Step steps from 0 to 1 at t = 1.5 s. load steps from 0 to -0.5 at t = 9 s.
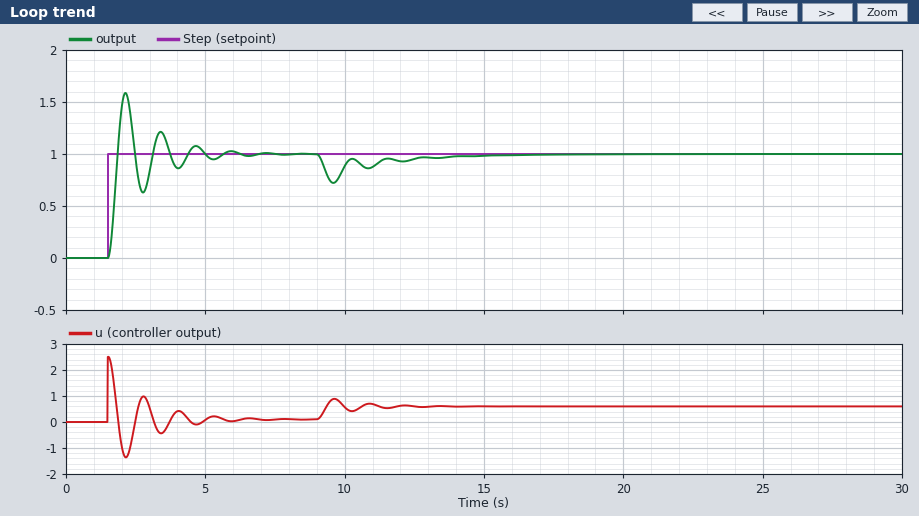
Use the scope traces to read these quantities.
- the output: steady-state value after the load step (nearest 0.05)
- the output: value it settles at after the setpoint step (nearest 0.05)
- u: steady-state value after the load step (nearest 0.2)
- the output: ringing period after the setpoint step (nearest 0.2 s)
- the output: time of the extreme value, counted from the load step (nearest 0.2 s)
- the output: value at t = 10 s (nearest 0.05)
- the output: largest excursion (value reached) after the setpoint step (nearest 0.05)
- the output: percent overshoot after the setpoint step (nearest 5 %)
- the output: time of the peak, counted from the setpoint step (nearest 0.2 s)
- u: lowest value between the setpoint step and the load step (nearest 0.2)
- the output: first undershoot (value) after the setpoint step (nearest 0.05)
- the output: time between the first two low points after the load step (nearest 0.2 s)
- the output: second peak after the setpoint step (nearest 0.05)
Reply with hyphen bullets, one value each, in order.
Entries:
- 1.00
- 1.00
- 0.6
- 1.2 s
- 0.6 s
- 0.90
- 1.60
- 60 %
- 0.6 s
- -1.4
- 0.65
- 1.2 s
- 1.20
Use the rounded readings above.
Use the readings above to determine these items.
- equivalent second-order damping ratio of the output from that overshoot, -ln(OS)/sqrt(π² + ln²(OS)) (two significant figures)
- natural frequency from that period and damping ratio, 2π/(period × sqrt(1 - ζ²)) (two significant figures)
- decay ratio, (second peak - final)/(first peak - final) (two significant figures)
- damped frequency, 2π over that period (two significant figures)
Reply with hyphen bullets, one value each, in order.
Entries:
- 0.16
- 5.3 rad/s
- 0.33
- 5.2 rad/s
